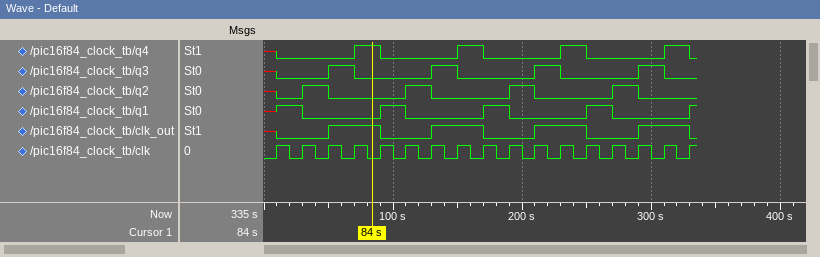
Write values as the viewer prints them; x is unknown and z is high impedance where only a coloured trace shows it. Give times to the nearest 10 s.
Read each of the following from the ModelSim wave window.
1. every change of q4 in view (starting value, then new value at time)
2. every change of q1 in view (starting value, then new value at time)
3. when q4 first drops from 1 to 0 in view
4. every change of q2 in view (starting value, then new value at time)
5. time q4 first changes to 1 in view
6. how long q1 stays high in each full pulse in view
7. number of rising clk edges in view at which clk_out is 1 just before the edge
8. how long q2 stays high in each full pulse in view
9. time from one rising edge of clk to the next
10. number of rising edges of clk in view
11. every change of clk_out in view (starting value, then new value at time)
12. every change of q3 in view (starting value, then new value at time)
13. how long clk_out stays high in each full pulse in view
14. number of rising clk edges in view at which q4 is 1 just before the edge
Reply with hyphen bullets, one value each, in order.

- x, 0 at 10 s, 1 at 70 s, 0 at 90 s, 1 at 150 s, 0 at 170 s, 1 at 230 s, 0 at 250 s, 1 at 310 s, 0 at 330 s
- x, 1 at 10 s, 0 at 30 s, 1 at 90 s, 0 at 110 s, 1 at 170 s, 0 at 190 s, 1 at 250 s, 0 at 270 s, 1 at 330 s
- 90 s
- x, 0 at 10 s, 1 at 30 s, 0 at 50 s, 1 at 110 s, 0 at 130 s, 1 at 190 s, 0 at 210 s, 1 at 270 s, 0 at 290 s
- 70 s
- 20 s, 20 s, 20 s
- 8
- 20 s, 20 s, 20 s, 20 s
- 20 s
- 17
- x, 0 at 10 s, 1 at 50 s, 0 at 90 s, 1 at 130 s, 0 at 170 s, 1 at 210 s, 0 at 250 s, 1 at 290 s, 0 at 330 s
- x, 0 at 10 s, 1 at 50 s, 0 at 70 s, 1 at 130 s, 0 at 150 s, 1 at 210 s, 0 at 230 s, 1 at 290 s, 0 at 310 s
- 40 s, 40 s, 40 s, 40 s
- 4
